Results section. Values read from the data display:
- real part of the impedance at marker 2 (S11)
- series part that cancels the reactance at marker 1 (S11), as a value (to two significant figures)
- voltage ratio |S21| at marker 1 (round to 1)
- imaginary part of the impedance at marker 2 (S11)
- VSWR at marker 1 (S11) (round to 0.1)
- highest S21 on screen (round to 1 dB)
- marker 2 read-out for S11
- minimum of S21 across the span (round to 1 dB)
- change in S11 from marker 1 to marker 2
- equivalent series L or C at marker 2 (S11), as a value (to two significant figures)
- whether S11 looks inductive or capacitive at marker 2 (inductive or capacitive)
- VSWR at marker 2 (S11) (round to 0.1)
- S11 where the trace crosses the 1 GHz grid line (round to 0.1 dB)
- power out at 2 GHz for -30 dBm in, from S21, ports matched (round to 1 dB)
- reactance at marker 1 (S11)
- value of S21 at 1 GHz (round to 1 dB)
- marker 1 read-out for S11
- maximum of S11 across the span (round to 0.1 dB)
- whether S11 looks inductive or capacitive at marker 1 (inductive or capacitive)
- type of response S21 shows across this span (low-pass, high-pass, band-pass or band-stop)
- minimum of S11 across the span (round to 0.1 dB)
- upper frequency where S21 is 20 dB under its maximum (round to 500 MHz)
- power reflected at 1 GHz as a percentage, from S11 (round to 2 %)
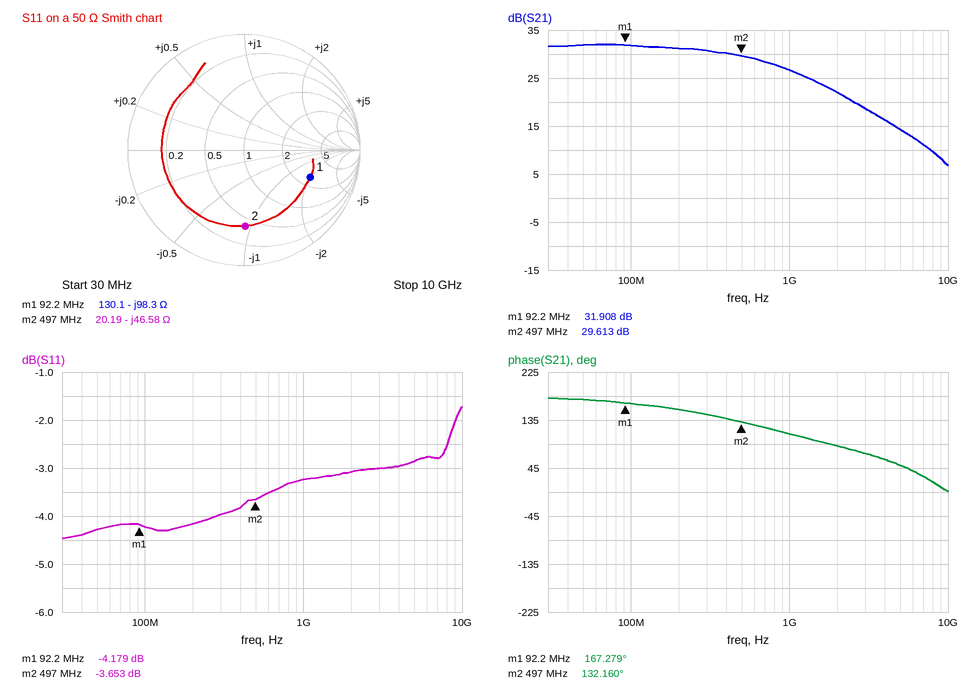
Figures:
20.19 Ω
170 nH
39
-46.58 Ω
4.2
32 dB
-3.653 dB
7 dB
0.526 dB
6.9 pF
capacitive
4.8
-3.2 dB
-8 dBm
-98.3 Ω
27 dB
-4.179 dB
-1.7 dB
capacitive
low-pass
-4.5 dB
6.5 GHz
48 %
